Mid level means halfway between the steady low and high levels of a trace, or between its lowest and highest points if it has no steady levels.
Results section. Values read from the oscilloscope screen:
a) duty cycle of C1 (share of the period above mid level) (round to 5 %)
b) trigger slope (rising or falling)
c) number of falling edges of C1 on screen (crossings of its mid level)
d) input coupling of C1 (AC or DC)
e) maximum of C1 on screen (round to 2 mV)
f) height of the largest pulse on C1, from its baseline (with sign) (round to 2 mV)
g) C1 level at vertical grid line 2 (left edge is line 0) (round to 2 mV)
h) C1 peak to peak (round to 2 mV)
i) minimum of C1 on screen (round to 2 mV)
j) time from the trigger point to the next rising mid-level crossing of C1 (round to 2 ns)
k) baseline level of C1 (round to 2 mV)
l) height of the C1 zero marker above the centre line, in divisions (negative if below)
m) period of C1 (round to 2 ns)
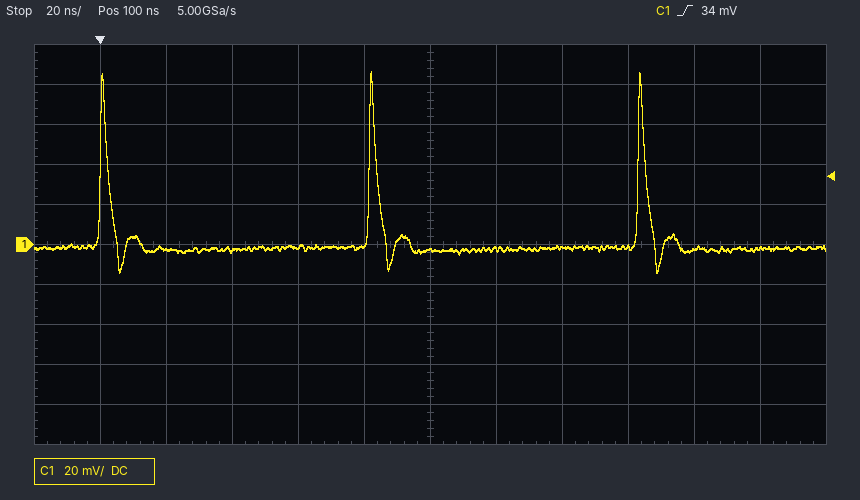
5 %
rising
3
DC
86 mV
+88 mV
-2 mV
100 mV
-14 mV
82 ns
-2 mV
0.0 div
82 ns
